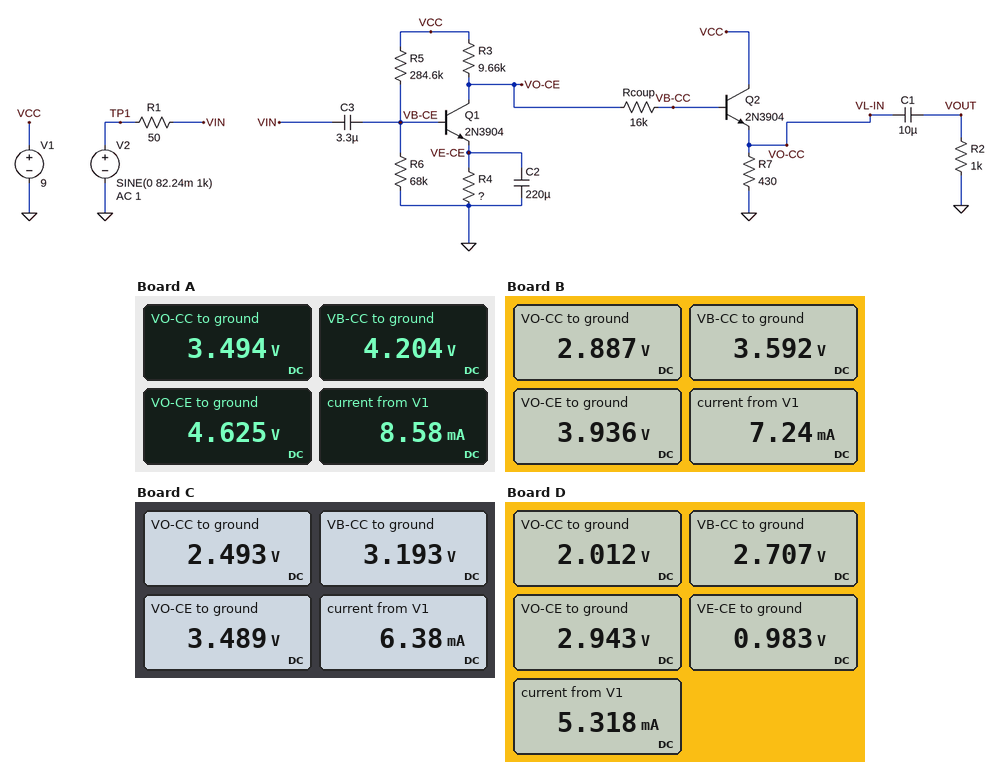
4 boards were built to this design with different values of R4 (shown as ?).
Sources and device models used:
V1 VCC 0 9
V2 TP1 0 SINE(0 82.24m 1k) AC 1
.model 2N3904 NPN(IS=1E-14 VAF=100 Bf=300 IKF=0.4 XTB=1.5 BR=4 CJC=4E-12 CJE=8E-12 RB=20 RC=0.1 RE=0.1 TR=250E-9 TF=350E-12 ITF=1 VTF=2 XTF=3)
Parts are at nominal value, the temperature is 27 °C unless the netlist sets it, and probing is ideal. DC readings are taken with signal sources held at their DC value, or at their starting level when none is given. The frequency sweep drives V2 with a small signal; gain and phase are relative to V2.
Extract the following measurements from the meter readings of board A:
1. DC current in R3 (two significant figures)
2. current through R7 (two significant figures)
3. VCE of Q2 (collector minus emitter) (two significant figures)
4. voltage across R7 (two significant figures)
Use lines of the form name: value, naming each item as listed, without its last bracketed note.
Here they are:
DC current in R3: 450 µA
current through R7: 8.1 mA
VCE of Q2 (collector minus emitter): 5.5 V
voltage across R7: 3.5 V
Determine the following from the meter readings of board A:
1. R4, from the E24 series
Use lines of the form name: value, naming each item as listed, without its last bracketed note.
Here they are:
R4, from the E24 series: 2.4 kΩ
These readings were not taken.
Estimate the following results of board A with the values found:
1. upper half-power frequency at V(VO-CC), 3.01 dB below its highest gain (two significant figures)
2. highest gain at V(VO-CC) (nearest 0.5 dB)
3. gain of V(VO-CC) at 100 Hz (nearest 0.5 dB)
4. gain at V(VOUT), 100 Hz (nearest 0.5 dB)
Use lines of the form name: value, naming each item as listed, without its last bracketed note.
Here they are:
upper half-power frequency at V(VO-CC), 3.01 dB below its highest gain: 1.7 MHz
highest gain at V(VO-CC): 41.5 dB
gain of V(VO-CC) at 100 Hz: 41.5 dB
gain at V(VOUT), 100 Hz: 41.0 dB
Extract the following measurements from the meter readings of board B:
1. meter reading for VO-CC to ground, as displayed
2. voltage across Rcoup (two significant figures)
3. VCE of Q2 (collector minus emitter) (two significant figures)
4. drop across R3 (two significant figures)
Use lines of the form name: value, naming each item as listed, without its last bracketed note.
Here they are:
meter reading for VO-CC to ground, as displayed: 2.887 V
voltage across Rcoup: 340 mV
VCE of Q2 (collector minus emitter): 6.1 V
drop across R3: 5.1 V
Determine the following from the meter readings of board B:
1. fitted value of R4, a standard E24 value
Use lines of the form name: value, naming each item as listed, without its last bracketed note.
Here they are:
fitted value of R4, a standard E24 value: 2 kΩ
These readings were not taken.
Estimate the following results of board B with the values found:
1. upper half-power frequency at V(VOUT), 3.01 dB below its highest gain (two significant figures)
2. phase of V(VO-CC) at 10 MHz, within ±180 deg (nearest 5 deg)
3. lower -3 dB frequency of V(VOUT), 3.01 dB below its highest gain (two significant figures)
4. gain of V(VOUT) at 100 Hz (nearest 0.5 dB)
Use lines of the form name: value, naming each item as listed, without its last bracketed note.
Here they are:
upper half-power frequency at V(VOUT), 3.01 dB below its highest gain: 1.6 MHz
phase of V(VO-CC) at 10 MHz, within ±180 deg: 40 deg
lower -3 dB frequency of V(VOUT), 3.01 dB below its highest gain: 25 Hz
gain of V(VOUT) at 100 Hz: 42.5 dB
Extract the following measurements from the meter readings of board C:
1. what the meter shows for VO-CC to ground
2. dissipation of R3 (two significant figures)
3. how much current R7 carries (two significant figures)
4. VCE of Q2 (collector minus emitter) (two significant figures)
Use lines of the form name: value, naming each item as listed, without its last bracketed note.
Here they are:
what the meter shows for VO-CC to ground: 2.493 V
dissipation of R3: 3.1 mW
how much current R7 carries: 5.8 mA
VCE of Q2 (collector minus emitter): 6.5 V
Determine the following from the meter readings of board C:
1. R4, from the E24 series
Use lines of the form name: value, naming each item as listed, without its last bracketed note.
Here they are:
R4, from the E24 series: 1.8 kΩ
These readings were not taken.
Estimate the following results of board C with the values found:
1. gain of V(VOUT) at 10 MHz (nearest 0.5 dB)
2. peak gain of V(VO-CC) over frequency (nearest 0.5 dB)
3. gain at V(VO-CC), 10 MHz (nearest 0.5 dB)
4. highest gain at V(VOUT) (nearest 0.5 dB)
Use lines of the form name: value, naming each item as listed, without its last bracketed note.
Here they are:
gain of V(VOUT) at 10 MHz: 22.0 dB
peak gain of V(VO-CC) over frequency: 43.5 dB
gain at V(VO-CC), 10 MHz: 22.0 dB
highest gain at V(VOUT): 43.5 dB
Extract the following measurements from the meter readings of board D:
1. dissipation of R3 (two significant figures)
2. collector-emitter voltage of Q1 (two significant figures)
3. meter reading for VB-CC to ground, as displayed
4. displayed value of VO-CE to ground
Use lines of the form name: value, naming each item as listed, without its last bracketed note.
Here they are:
dissipation of R3: 3.8 mW
collector-emitter voltage of Q1: 2.0 V
meter reading for VB-CC to ground, as displayed: 2.707 V
displayed value of VO-CE to ground: 2.943 V
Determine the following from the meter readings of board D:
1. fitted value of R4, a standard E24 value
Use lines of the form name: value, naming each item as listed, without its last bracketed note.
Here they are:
fitted value of R4, a standard E24 value: 1.6 kΩ
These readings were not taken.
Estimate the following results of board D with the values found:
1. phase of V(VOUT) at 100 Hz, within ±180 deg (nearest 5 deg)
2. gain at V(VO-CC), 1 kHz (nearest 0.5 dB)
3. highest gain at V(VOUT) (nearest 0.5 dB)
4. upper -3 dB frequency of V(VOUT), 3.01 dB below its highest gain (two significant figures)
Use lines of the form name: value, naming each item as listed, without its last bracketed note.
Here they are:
phase of V(VOUT) at 100 Hz, within ±180 deg: -160 deg
gain at V(VO-CC), 1 kHz: 44.5 dB
highest gain at V(VOUT): 44.5 dB
upper -3 dB frequency of V(VOUT), 3.01 dB below its highest gain: 1.5 MHz
